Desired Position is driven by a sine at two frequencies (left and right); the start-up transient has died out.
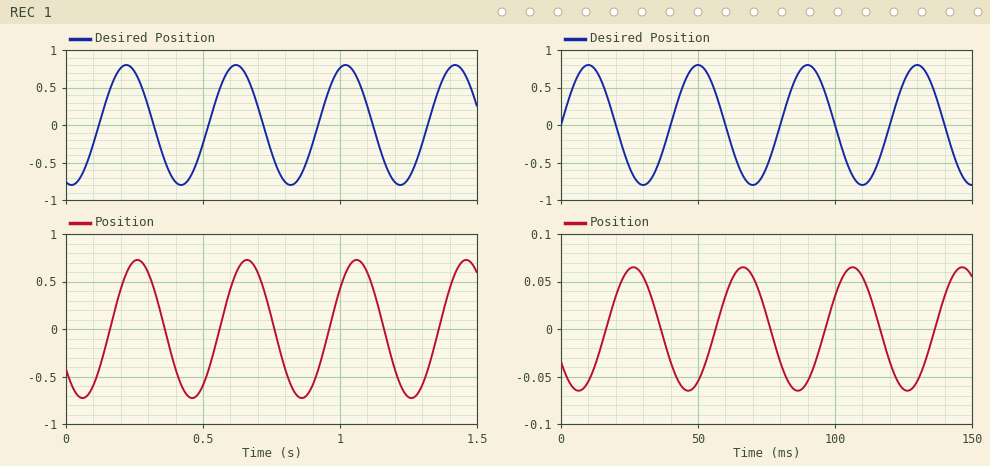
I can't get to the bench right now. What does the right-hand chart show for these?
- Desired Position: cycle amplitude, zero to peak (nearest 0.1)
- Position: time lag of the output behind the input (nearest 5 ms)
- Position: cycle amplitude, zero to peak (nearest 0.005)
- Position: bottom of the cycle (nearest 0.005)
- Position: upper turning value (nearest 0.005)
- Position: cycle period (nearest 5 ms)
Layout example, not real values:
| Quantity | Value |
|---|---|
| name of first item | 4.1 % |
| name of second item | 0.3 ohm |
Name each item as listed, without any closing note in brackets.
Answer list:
| Quantity | Value |
|---|---|
| Desired Position: cycle amplitude, zero to peak | 0.8 |
| Position: time lag of the output behind the input | 15 ms |
| Position: cycle amplitude, zero to peak | 0.065 |
| Position: bottom of the cycle | -0.065 |
| Position: upper turning value | 0.065 |
| Position: cycle period | 40 ms |
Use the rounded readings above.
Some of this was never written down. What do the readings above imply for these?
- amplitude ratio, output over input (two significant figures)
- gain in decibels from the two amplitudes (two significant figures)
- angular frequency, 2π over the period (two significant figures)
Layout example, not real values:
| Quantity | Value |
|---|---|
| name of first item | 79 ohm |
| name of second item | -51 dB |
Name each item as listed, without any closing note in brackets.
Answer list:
| Quantity | Value |
|---|---|
| amplitude ratio, output over input | 0.081 |
| gain in decibels from the two amplitudes | -22 dB |
| angular frequency, 2π over the period | 0.16 rad/ms |
